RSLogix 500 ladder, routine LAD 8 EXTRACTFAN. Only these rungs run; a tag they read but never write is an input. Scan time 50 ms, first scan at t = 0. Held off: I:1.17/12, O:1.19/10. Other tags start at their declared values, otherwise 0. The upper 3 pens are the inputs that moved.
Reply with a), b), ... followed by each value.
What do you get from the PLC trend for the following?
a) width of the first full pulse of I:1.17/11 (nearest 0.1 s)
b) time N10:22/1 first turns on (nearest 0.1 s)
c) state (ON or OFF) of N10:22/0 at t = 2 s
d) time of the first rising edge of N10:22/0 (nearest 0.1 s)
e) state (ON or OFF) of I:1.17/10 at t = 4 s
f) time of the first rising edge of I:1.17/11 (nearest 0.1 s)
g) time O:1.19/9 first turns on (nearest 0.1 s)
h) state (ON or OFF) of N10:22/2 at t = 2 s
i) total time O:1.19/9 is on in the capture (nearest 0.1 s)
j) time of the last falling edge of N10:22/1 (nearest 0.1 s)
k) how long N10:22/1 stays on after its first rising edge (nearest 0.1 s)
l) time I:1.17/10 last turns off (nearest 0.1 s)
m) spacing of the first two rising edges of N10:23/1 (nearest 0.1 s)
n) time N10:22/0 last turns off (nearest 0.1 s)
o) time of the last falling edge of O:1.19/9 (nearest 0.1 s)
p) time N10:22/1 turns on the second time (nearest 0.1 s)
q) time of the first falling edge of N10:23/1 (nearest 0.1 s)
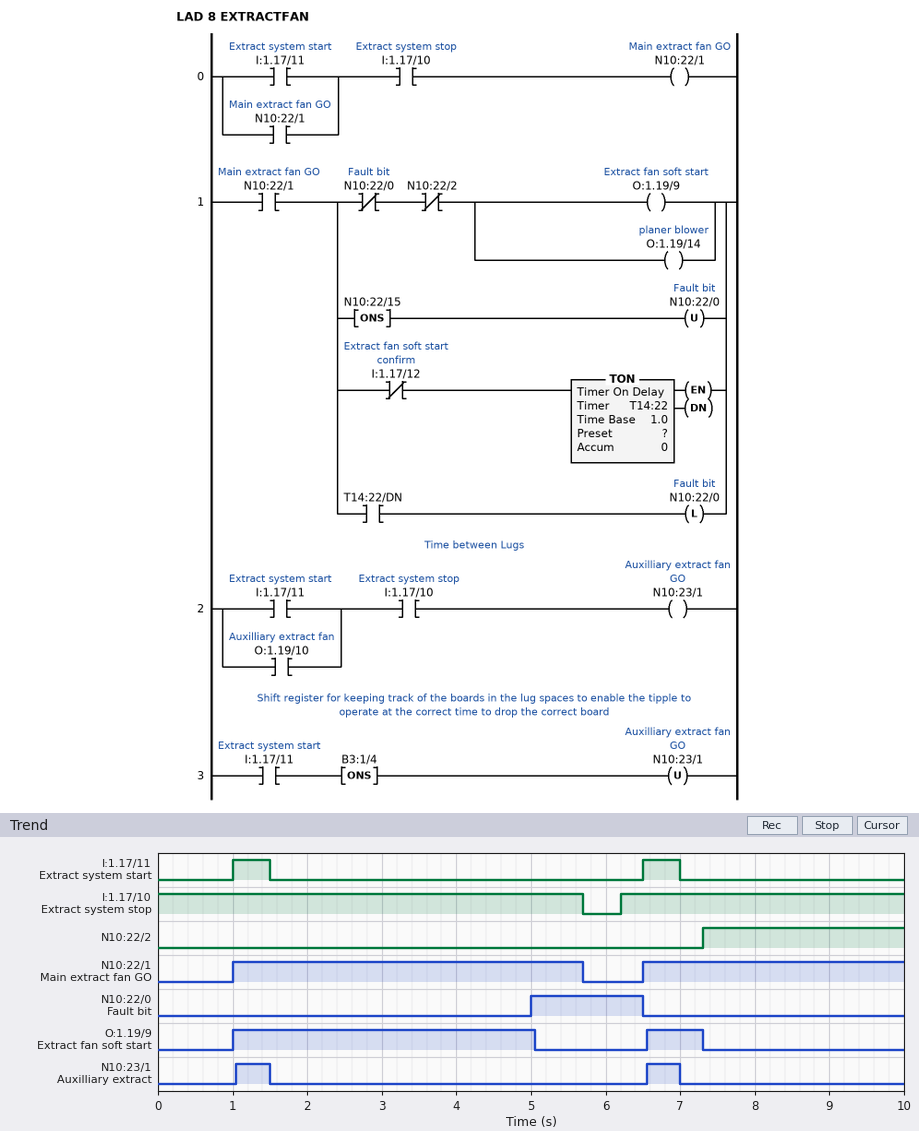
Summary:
a) 0.5 s
b) 1.0 s
c) OFF
d) 5.0 s
e) ON
f) 1.0 s
g) 1.0 s
h) OFF
i) 4.8 s
j) 5.7 s
k) 4.7 s
l) 5.7 s
m) 5.5 s
n) 6.5 s
o) 7.3 s
p) 6.5 s
q) 1.5 s
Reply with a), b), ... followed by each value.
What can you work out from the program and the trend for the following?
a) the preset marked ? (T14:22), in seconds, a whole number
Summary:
a) 4 s
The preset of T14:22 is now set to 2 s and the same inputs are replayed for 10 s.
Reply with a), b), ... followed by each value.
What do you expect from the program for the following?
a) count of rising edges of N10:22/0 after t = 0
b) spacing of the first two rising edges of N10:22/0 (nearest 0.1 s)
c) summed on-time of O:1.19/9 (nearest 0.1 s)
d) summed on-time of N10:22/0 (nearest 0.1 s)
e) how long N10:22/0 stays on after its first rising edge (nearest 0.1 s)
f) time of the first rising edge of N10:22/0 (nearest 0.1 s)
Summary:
a) 2
b) 5.5 s
c) 2.8 s
d) 5.0 s
e) 3.5 s
f) 3.0 s
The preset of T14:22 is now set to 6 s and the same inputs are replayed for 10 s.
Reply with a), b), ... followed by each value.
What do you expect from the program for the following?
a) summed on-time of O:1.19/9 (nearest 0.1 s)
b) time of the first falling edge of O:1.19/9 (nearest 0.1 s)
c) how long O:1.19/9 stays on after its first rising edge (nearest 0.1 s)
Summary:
a) 5.5 s
b) 5.7 s
c) 4.7 s
